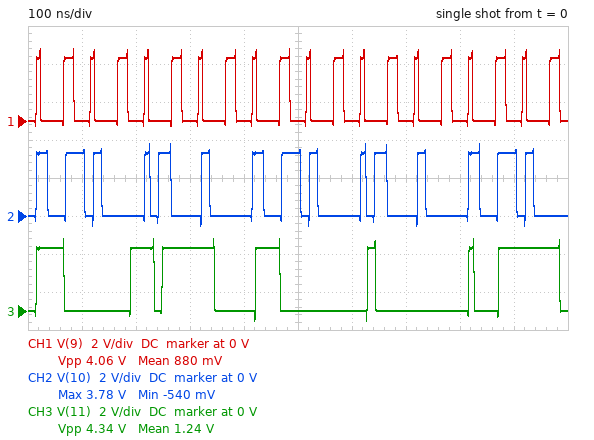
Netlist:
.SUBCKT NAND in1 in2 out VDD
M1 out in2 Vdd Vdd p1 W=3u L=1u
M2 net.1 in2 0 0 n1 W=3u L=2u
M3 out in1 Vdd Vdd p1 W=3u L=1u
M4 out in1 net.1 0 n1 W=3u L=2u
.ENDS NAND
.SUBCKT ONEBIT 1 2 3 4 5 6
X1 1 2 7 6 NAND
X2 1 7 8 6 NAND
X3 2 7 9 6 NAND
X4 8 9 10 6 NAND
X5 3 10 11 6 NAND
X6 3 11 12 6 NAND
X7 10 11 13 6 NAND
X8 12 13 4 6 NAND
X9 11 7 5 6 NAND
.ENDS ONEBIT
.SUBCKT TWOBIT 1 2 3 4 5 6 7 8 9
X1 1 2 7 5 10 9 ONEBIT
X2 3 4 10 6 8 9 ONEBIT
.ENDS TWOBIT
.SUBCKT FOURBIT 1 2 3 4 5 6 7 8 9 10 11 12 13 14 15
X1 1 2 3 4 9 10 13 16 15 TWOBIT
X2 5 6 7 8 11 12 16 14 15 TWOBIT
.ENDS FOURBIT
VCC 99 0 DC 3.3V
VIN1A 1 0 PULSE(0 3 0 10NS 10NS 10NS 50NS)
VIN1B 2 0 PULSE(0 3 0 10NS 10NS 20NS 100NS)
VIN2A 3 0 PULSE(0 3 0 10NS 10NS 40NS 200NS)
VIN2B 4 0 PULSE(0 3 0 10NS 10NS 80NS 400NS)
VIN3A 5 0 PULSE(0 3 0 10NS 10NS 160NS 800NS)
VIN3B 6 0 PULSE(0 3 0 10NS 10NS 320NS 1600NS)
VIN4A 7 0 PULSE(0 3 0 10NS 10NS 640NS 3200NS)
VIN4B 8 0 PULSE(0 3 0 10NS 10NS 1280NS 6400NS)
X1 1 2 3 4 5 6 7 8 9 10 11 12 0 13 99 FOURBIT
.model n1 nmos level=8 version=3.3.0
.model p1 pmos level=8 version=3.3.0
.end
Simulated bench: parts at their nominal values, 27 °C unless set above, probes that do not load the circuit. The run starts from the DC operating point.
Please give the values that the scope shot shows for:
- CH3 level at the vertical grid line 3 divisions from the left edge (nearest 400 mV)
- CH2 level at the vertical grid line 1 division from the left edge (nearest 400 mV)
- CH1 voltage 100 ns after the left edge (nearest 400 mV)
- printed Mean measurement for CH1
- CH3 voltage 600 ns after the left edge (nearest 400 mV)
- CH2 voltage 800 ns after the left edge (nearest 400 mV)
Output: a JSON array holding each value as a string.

["3.2 V", "3.2 V", "0 V", "880 mV", "0 V", "0 V"]
